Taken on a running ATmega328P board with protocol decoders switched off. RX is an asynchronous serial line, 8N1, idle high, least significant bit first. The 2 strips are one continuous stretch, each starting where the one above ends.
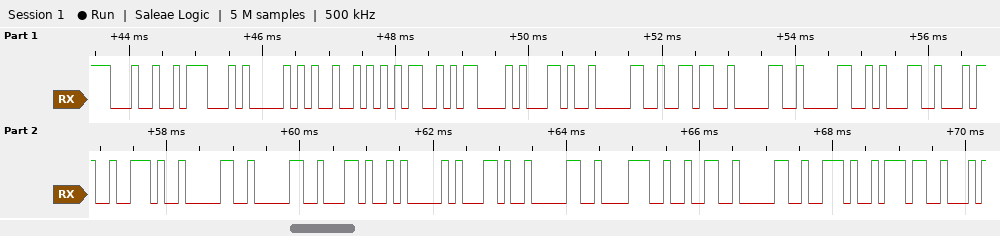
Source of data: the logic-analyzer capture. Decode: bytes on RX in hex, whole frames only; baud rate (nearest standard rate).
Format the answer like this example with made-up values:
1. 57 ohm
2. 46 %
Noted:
1. 0x24 0x47 0x50 0x52 0x4D 0x43 0x2C 0x30 0x36 0x30 0x30 0x31 0x34 0x2E 0x30 0x30 0x2C 0x41 0x2C 0x30 0x38 0x32 0x30 0x2E 0x37
2. 9600 baud
